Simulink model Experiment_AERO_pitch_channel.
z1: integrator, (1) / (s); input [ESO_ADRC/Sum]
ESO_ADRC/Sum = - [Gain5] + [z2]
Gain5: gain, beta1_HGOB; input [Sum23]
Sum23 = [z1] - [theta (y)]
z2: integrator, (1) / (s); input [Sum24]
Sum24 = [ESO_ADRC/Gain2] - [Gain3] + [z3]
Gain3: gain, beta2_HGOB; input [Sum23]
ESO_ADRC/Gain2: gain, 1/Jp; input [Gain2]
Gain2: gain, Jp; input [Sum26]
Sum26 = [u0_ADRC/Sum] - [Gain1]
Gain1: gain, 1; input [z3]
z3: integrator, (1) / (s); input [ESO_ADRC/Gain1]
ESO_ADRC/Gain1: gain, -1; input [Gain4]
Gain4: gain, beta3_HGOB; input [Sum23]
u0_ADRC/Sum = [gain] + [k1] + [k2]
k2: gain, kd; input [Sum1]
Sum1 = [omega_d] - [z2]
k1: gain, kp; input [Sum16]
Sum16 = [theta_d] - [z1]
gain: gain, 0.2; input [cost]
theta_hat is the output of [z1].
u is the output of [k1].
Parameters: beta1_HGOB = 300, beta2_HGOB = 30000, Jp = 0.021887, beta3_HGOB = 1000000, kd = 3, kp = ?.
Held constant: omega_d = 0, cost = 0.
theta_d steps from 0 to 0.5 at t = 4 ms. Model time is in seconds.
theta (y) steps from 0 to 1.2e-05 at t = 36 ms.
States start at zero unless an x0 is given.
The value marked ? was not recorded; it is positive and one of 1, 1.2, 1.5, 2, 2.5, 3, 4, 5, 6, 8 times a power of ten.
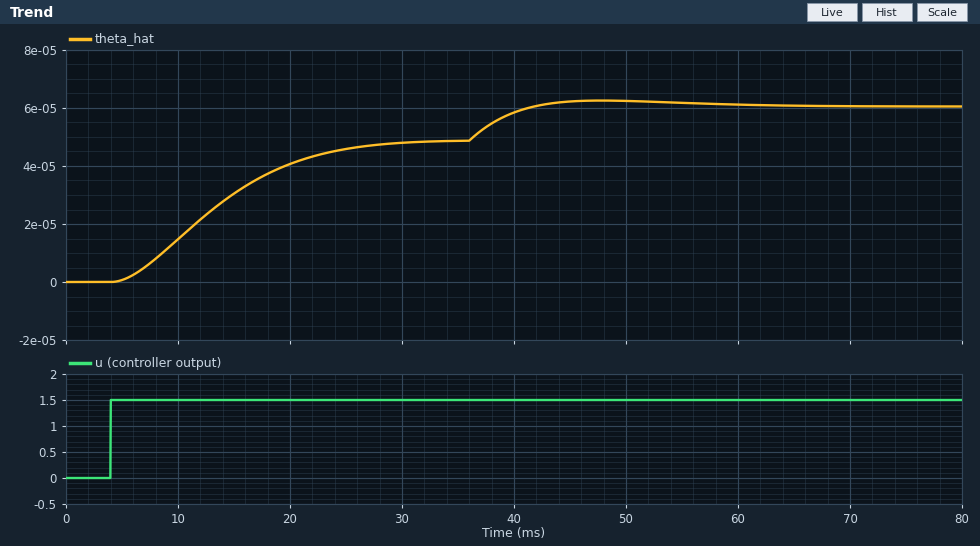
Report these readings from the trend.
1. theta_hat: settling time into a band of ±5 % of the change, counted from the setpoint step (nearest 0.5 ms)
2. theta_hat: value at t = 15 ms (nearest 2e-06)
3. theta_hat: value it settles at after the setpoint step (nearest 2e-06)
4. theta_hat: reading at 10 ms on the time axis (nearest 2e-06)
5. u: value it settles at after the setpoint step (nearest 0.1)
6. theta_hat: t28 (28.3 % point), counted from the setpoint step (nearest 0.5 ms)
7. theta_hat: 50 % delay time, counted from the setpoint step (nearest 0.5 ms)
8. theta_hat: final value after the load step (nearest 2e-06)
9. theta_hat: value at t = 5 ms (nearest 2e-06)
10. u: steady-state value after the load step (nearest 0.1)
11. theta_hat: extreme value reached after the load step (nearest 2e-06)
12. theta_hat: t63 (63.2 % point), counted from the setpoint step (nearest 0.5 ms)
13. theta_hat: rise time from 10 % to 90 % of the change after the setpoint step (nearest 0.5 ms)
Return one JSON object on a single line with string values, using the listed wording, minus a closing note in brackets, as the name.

{"theta_hat: settling time into a band of ±5 % of the change, counted from the setpoint step": "21.5 ms", "theta_hat: value at t = 15 ms": "0.000030", "theta_hat: value it settles at after the setpoint step": "0.000048", "theta_hat: reading at 10 ms on the time axis": "0.000014", "u: value it settles at after the setpoint step": "1.5", "theta_hat: t28 (28.3 % point), counted from the setpoint step": "5.5 ms", "theta_hat: 50 % delay time, counted from the setpoint step": "9.0 ms", "theta_hat: final value after the load step": "0.000060", "theta_hat: value at t = 5 ms": "0.000000", "u: steady-state value after the load step": "1.5", "theta_hat: extreme value reached after the load step": "0.000062", "theta_hat: t63 (63.2 % point), counted from the setpoint step": "11.0 ms", "theta_hat: rise time from 10 % to 90 % of the change after the setpoint step": "15.5 ms"}
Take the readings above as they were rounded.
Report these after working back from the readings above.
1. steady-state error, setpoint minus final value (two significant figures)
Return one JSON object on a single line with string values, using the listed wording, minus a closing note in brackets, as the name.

{"steady-state error, setpoint minus final value": "0.50"}
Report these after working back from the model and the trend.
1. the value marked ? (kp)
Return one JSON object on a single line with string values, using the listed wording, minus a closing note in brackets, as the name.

{"the value marked ?": "3"}
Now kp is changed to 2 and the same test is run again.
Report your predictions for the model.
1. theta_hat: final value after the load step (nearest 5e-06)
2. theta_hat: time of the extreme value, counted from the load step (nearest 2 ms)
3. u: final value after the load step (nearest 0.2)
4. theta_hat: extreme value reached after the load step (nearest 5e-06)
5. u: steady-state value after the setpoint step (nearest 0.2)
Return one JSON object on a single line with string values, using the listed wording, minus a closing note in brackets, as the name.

{"theta_hat: final value after the load step": "0.000045", "theta_hat: time of the extreme value, counted from the load step": "12 ms", "u: final value after the load step": "1.0", "theta_hat: extreme value reached after the load step": "0.000045", "u: steady-state value after the setpoint step": "1.0"}
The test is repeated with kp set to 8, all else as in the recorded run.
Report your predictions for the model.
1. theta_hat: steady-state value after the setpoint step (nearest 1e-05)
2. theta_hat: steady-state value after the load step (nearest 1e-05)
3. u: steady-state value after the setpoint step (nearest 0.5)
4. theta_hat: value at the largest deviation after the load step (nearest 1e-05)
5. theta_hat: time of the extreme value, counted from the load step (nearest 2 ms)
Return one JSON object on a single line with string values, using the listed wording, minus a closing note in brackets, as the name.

{"theta_hat: steady-state value after the setpoint step": "0.00013", "theta_hat: steady-state value after the load step": "0.00014", "u: steady-state value after the setpoint step": "4.0", "theta_hat: value at the largest deviation after the load step": "0.00014", "theta_hat: time of the extreme value, counted from the load step": "12 ms"}
